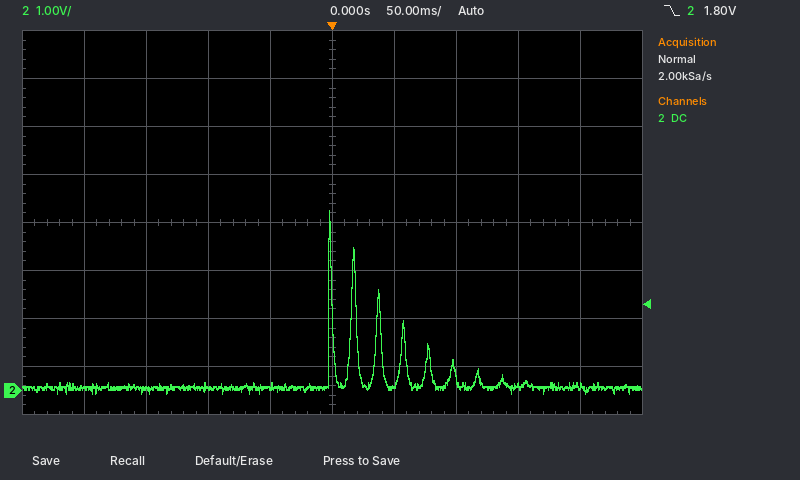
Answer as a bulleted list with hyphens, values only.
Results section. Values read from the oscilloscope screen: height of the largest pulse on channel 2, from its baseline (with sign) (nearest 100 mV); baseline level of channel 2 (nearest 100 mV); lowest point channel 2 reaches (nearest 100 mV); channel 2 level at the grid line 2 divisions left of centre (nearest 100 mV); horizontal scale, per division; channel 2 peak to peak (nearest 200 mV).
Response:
- +3.7 V
- 100 mV
- -100 mV
- 100 mV
- 50 ms
- 3.8 V
